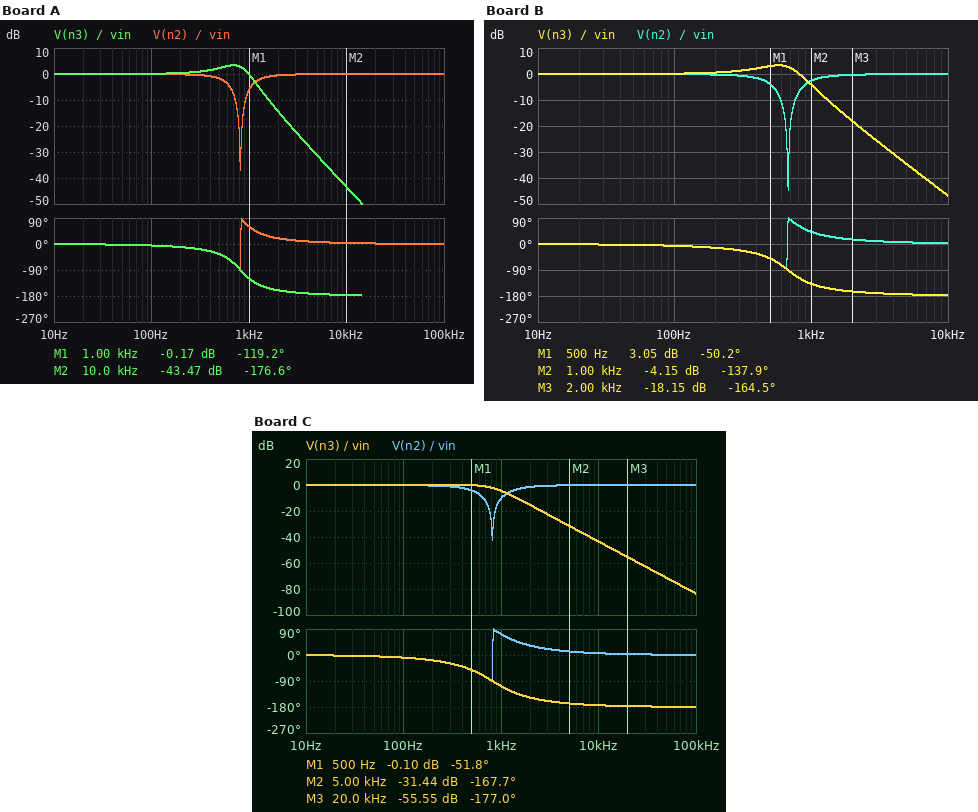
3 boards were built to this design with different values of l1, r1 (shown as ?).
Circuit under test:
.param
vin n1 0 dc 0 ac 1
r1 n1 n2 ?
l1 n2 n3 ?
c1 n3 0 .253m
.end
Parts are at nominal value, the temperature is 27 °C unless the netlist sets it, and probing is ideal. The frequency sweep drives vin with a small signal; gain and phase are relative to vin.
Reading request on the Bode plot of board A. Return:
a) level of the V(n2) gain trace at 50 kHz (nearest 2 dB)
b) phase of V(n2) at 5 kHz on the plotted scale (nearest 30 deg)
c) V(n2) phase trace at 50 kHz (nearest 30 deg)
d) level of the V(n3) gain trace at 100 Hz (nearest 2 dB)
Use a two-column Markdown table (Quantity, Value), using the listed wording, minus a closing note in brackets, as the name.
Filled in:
| Quantity | Value |
|---|---|
| level of the V(n2) gain trace at 50 kHz | 0 dB |
| phase of V(n2) at 5 kHz on the plotted scale | 0 deg |
| V(n2) phase trace at 50 kHz | 0 deg |
| level of the V(n3) gain trace at 100 Hz | 0 dB |
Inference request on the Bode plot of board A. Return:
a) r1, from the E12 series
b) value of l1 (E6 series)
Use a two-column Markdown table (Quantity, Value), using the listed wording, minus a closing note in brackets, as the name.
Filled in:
| Quantity | Value |
|---|---|
| r1, from the E12 series | 0.56 Ω |
| value of l1 | 150 µH |
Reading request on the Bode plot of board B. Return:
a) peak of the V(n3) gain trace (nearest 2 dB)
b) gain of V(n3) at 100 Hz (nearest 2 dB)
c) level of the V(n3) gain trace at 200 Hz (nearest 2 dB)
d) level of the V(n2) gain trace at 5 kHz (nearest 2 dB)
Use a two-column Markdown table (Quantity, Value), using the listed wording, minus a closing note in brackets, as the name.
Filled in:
| Quantity | Value |
|---|---|
| peak of the V(n3) gain trace | 4 dB |
| gain of V(n3) at 100 Hz | 0 dB |
| level of the V(n3) gain trace at 200 Hz | 0 dB |
| level of the V(n2) gain trace at 5 kHz | 0 dB |
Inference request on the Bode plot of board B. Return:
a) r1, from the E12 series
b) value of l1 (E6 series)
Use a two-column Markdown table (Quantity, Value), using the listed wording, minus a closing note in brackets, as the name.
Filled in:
| Quantity | Value |
|---|---|
| r1, from the E12 series | 0.68 Ω |
| value of l1 | 220 µH |
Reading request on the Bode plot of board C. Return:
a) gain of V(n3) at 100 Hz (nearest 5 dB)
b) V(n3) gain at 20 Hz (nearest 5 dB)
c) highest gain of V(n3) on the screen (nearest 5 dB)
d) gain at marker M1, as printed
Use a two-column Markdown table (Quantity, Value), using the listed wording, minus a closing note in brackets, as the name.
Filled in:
| Quantity | Value |
|---|---|
| gain of V(n3) at 100 Hz | 0 dB |
| V(n3) gain at 20 Hz | 0 dB |
| highest gain of V(n3) on the screen | 0 dB |
| gain at marker M1, as printed | -0.10 dB |
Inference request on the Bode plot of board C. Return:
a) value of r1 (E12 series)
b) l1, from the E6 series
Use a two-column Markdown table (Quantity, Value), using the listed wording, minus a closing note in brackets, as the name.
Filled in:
| Quantity | Value |
|---|---|
| value of r1 | 1 Ω |
| l1, from the E6 series | 150 µH |
